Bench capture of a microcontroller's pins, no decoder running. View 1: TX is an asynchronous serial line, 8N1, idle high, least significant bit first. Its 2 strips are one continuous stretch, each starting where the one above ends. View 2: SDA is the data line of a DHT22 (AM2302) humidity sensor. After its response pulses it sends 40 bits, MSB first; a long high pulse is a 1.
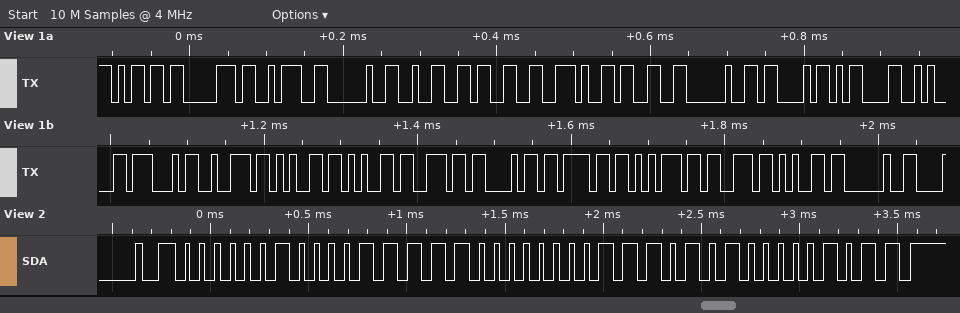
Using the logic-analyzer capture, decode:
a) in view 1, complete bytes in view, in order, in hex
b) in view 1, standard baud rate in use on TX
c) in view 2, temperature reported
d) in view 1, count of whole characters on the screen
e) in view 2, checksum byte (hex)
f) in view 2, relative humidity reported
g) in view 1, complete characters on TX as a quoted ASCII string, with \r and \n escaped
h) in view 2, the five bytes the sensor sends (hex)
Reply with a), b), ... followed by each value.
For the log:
a) 6D 70 3A 20 32 33 2E 33 20 43 0D 0A 47 72 65 65 6E 68 6F 75 73 65 20
b) 115200 baud
c) 23.4 °C
d) 23
e) 0x0B
f) 54.3 %
g) "mp: 23.3 C\r\nGreenhouse "
h) 02 1F 00 EA 0B
